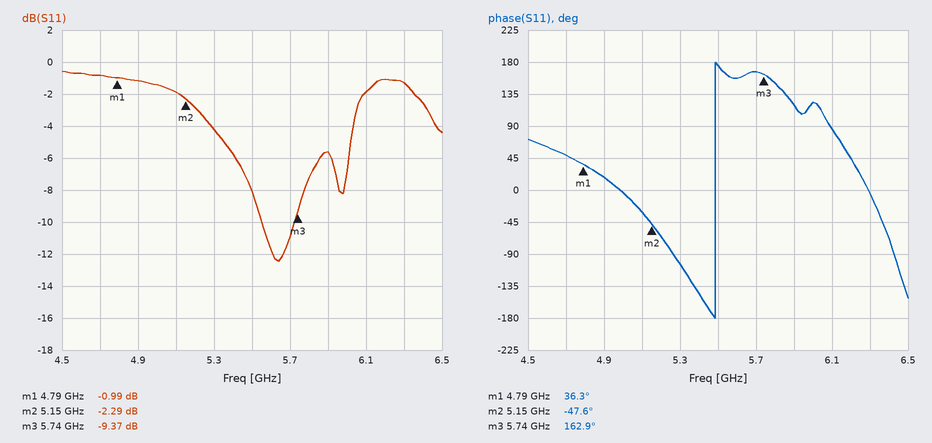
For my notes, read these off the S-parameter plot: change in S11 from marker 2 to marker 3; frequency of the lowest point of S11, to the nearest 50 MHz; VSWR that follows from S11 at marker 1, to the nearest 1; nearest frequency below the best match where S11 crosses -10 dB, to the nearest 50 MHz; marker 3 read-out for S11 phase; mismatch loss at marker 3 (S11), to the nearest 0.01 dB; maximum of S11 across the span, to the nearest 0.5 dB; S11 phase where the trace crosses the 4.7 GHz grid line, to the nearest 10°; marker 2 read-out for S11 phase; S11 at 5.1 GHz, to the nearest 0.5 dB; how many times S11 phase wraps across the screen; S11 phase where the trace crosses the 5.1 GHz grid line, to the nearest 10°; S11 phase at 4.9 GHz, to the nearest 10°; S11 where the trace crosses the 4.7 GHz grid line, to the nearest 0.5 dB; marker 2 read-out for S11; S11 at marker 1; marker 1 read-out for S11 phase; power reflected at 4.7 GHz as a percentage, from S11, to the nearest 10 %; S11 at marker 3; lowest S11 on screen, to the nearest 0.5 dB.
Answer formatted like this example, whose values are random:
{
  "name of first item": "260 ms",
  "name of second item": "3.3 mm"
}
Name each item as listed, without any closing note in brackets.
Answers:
{
  "change in S11 from marker 2 to marker 3": "-7.08 dB",
  "frequency of the lowest point of S11, to the nearest 50 MHz": "5.65 GHz",
  "VSWR that follows from S11 at marker 1, to the nearest 1": "18",
  "nearest frequency below the best match where S11 crosses -10 dB, to the nearest 50 MHz": "5.55 GHz",
  "marker 3 read-out for S11 phase": "162.9°",
  "mismatch loss at marker 3 (S11), to the nearest 0.01 dB": "0.53 dB",
  "maximum of S11 across the span, to the nearest 0.5 dB": "-0.5 dB",
  "S11 phase where the trace crosses the 4.7 GHz grid line, to the nearest 10°": "50°",
  "marker 2 read-out for S11 phase": "-47.6°",
  "S11 at 5.1 GHz, to the nearest 0.5 dB": "-2.0 dB",
  "how many times S11 phase wraps across the screen": "1",
  "S11 phase where the trace crosses the 5.1 GHz grid line, to the nearest 10°": "-30°",
  "S11 phase at 4.9 GHz, to the nearest 10°": "20°",
  "S11 where the trace crosses the 4.7 GHz grid line, to the nearest 0.5 dB": "-1.0 dB",
  "marker 2 read-out for S11": "-2.29 dB",
  "S11 at marker 1": "-0.99 dB",
  "marker 1 read-out for S11 phase": "36.3°",
  "power reflected at 4.7 GHz as a percentage, from S11, to the nearest 10 %": "80 %",
  "S11 at marker 3": "-9.37 dB",
  "lowest S11 on screen, to the nearest 0.5 dB": "-12.5 dB"
}
